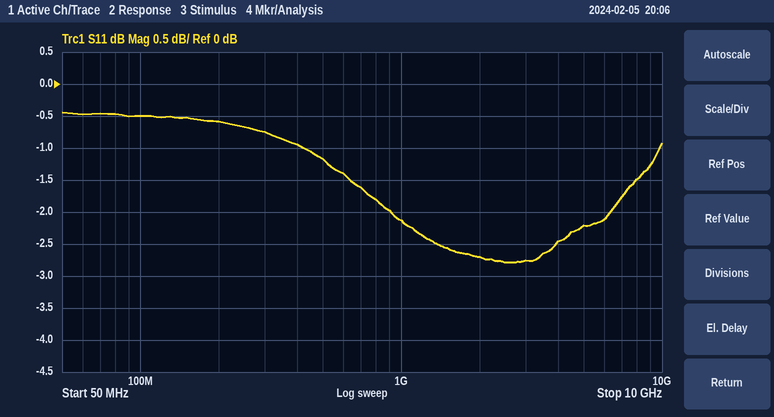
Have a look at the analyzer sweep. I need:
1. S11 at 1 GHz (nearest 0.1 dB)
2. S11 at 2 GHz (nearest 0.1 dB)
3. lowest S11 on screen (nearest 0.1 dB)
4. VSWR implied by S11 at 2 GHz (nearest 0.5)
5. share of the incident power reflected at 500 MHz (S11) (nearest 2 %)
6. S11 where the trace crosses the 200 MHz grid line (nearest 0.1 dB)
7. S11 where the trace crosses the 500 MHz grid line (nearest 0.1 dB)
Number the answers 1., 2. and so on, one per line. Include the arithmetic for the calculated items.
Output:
1. -2.1 dB
2. -2.7 dB
3. -2.8 dB
4. |Γ| = 10^(-2.7/20) = 0.7328; VSWR = (1 + 0.7328)/(1 − 0.7328) ≈ 6.5
5. 10^(-1.2/10) ≈ 76 %
6. -0.6 dB
7. -1.2 dB
